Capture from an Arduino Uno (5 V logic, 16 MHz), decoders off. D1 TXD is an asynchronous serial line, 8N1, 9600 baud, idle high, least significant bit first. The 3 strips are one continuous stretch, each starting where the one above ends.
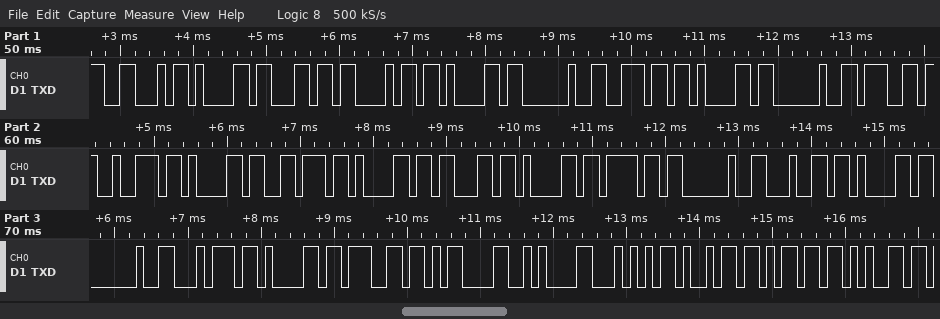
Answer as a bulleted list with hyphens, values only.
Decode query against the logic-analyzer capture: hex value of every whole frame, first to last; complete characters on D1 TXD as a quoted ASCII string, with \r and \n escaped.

- 46 61 6C 68 61 20 6E 61 20 67 72 61 76 61 63 61 6F 20 64 61 20 74 61 67 0D 0A 54 69 6D 65
- "Falha na gravacao da tag\r\nTime"
